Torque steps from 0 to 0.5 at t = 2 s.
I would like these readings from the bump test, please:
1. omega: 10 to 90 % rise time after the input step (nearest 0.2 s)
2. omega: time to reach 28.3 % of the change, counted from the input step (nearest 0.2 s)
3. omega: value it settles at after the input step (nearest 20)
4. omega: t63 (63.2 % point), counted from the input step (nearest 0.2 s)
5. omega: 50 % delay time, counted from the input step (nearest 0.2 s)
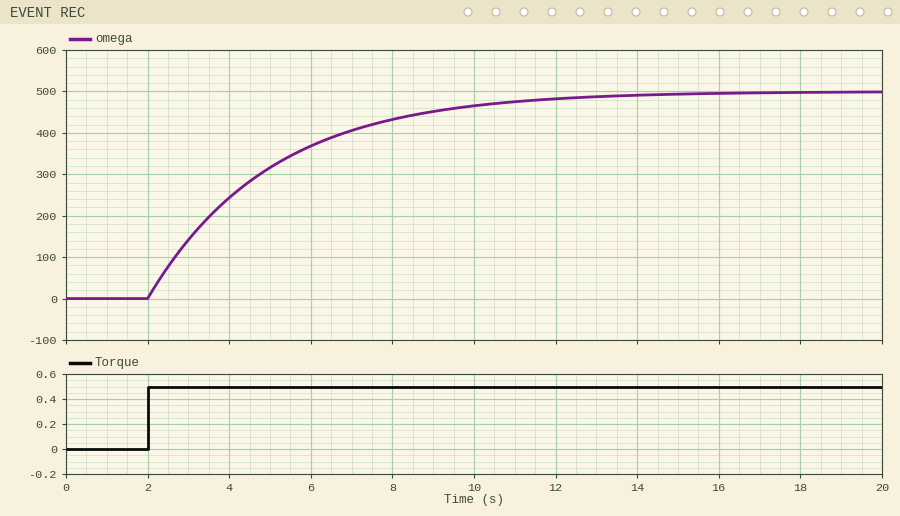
6.6 s
1.0 s
500
3.0 s
2.0 s
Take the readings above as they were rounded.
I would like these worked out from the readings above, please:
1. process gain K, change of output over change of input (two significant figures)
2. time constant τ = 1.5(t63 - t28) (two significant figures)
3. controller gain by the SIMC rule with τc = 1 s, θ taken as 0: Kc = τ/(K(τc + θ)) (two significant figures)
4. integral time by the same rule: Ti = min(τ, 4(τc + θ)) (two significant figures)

1000
3.0 s
0.0030
3.0 s
